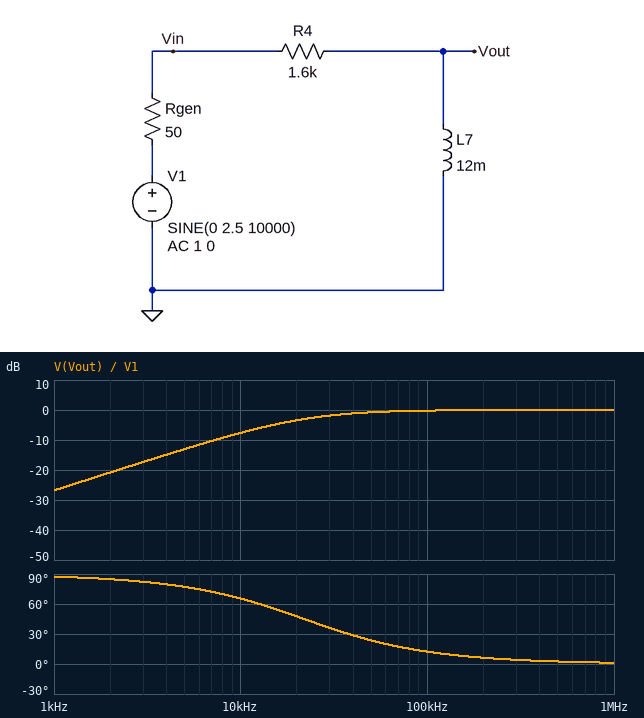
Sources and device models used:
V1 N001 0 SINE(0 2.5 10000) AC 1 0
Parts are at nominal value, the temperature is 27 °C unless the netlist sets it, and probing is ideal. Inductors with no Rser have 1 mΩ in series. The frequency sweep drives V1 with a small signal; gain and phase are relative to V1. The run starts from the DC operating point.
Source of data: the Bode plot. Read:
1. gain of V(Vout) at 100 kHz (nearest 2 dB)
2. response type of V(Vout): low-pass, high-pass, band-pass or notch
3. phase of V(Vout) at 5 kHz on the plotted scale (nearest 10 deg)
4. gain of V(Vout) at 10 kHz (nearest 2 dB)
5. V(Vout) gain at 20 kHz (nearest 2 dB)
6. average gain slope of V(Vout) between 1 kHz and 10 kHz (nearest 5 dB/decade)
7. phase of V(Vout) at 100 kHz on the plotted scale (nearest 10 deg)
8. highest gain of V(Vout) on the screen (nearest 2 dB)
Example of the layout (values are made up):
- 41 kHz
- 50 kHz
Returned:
- 0 dB
- high-pass
- 80 deg
- -8 dB
- -4 dB
- 20 dB/decade
- 10 deg
- 0 dB
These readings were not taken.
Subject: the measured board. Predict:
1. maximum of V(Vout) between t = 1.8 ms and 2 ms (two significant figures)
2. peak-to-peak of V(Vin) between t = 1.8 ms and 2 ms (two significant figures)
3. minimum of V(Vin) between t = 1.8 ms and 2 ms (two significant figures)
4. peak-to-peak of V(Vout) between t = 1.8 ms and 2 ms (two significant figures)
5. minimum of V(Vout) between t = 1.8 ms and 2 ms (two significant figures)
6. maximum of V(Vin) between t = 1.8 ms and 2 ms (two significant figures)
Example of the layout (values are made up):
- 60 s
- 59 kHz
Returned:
- 1.0 V
- 4.9 V
- -2.4 V
- 2.1 V
- -1.0 V
- 2.4 V
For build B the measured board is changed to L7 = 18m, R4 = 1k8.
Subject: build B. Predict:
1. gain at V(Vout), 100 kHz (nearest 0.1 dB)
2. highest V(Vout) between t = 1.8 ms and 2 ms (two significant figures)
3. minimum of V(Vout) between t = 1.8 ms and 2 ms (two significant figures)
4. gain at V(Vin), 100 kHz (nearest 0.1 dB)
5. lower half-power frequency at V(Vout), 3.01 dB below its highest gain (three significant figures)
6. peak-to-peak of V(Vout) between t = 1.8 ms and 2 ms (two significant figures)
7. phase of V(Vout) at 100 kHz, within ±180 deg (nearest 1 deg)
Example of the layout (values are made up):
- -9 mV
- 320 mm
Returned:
- -0.1 dB
- 1.3 V
- -1.3 V
- 0 dB
- 16.4 kHz
- 2.6 V
- 9 deg
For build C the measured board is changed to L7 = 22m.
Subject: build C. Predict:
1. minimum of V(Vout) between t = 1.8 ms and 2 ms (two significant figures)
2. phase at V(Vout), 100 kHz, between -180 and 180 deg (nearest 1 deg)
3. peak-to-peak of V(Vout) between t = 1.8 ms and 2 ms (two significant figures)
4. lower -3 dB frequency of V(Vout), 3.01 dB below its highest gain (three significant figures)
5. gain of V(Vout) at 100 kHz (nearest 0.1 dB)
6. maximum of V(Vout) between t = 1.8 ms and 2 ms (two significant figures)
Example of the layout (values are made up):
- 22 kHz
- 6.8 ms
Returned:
- -1.6 V
- 7 deg
- 3.2 V
- 11.9 kHz
- -0.1 dB
- 1.6 V
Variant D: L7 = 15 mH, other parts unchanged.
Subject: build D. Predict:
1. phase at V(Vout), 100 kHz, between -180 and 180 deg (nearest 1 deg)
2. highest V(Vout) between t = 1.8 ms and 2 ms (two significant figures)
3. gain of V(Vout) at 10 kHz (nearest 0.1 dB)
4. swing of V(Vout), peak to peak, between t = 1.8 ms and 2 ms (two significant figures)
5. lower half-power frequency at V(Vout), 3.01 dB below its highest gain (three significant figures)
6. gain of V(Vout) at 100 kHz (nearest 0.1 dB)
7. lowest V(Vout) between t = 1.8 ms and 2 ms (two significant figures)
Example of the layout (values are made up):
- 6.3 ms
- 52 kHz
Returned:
- 10 deg
- 1.2 V
- -6.1 dB
- 2.5 V
- 17.5 kHz
- -0.1 dB
- -1.2 V
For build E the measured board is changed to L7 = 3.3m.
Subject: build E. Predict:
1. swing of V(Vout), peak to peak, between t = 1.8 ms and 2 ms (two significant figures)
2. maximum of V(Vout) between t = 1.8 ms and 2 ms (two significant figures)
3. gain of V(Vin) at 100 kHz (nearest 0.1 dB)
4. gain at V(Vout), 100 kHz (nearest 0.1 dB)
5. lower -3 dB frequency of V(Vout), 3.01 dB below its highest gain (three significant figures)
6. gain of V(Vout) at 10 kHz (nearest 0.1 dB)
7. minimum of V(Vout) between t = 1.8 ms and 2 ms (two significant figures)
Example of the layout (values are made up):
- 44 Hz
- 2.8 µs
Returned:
- 620 mV
- 310 mV
- -0.1 dB
- -2.1 dB
- 79.6 kHz
- -18.1 dB
- -310 mV
